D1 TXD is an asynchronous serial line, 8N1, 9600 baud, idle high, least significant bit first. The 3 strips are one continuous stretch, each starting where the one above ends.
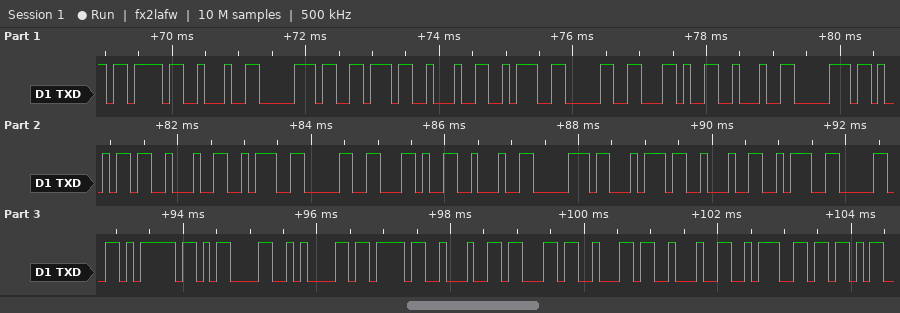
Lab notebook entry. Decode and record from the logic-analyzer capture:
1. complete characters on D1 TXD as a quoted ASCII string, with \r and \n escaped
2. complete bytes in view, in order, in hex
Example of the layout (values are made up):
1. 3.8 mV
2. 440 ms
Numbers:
1. "{\"pv\":0,\"pi\":0,\"pt\":0}\r\n{\"cb\":["
2. 7B 22 70 76 22 3A 30 2C 22 70 69 22 3A 30 2C 22 70 74 22 3A 30 7D 0D 0A 7B 22 63 62 22 3A 5B
